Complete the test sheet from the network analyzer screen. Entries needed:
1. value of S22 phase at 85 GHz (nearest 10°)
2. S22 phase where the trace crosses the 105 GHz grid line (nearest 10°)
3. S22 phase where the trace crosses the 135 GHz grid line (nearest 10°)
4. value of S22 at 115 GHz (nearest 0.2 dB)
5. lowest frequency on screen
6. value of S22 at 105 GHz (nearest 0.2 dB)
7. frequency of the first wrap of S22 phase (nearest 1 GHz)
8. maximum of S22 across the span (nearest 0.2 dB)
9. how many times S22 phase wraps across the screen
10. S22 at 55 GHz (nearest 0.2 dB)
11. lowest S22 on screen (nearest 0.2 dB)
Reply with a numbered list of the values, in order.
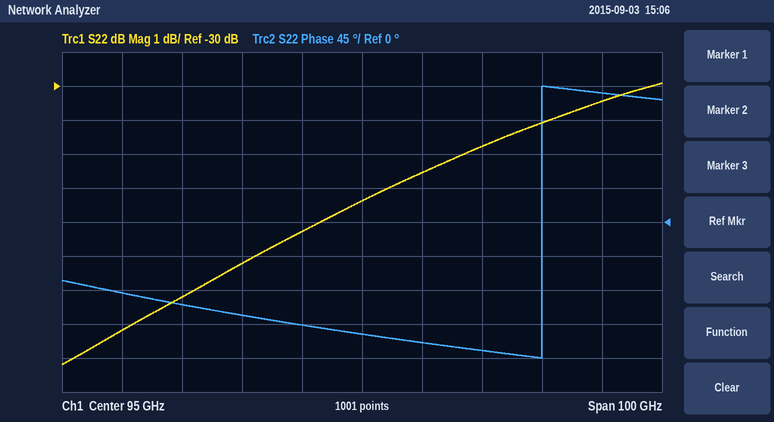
1. -140°
2. -160°
3. 170°
4. -31.8 dB
5. 45 GHz
6. -32.6 dB
7. 125 GHz
8. -30.0 dB
9. 1
10. -37.2 dB
11. -38.2 dB
